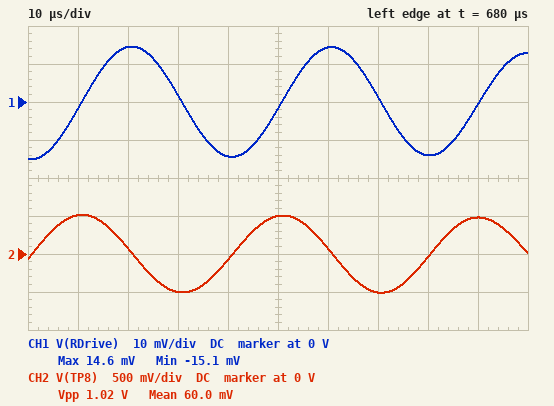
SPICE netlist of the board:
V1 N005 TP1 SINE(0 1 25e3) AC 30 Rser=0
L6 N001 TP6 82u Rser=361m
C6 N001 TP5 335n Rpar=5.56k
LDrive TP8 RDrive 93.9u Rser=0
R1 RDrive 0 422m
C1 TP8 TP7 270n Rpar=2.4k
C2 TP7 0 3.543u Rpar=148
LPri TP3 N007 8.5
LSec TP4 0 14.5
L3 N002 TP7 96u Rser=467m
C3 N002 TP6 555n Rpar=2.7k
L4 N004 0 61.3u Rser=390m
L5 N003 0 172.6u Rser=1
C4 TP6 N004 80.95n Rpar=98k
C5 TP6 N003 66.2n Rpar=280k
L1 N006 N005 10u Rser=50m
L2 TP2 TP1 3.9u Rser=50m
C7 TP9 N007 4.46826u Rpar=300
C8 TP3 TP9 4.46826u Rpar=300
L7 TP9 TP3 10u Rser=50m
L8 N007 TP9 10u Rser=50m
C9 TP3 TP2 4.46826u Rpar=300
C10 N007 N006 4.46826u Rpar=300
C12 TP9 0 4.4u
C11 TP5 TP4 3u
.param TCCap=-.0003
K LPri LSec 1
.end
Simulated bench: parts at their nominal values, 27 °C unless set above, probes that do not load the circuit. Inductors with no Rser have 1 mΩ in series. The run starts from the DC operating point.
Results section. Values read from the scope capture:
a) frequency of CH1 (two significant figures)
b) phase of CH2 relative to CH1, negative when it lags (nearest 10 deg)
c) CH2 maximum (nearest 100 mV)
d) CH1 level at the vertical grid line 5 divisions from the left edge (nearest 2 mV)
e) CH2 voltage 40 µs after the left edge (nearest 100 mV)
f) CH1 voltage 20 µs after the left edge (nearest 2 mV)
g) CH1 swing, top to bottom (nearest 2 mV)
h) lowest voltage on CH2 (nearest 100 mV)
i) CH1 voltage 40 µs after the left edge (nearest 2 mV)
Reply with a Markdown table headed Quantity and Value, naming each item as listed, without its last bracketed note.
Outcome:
| Quantity | Value |
|---|---|
| frequency of CH1 | 25 kHz |
| phase of CH2 relative to CH1, negative when it lags | 90 deg |
| CH2 maximum | 500 mV |
| CH1 level at the vertical grid line 5 divisions from the left edge | -2 mV |
| CH2 voltage 40 µs after the left edge | -100 mV |
| CH1 voltage 20 µs after the left edge | 14 mV |
| CH1 swing, top to bottom | 30 mV |
| lowest voltage on CH2 | -500 mV |
| CH1 voltage 40 µs after the left edge | -14 mV |
